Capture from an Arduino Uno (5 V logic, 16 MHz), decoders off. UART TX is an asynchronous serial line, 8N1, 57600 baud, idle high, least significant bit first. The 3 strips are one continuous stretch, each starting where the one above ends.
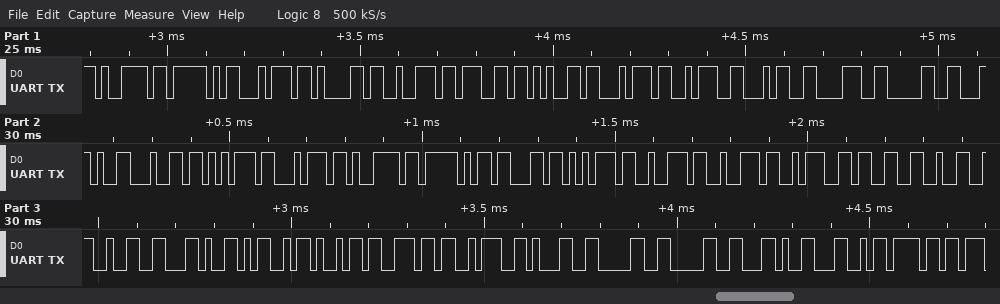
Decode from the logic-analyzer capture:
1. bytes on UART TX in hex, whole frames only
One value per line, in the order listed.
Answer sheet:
79 5F 74 61 72 67 65 74 3A 34 38 30 2C 64 75 74 79 5F 63 75 72 72 3A 33 32 32 2C 4D 69 6E 3A 31 30 30 2C 4C 6F
